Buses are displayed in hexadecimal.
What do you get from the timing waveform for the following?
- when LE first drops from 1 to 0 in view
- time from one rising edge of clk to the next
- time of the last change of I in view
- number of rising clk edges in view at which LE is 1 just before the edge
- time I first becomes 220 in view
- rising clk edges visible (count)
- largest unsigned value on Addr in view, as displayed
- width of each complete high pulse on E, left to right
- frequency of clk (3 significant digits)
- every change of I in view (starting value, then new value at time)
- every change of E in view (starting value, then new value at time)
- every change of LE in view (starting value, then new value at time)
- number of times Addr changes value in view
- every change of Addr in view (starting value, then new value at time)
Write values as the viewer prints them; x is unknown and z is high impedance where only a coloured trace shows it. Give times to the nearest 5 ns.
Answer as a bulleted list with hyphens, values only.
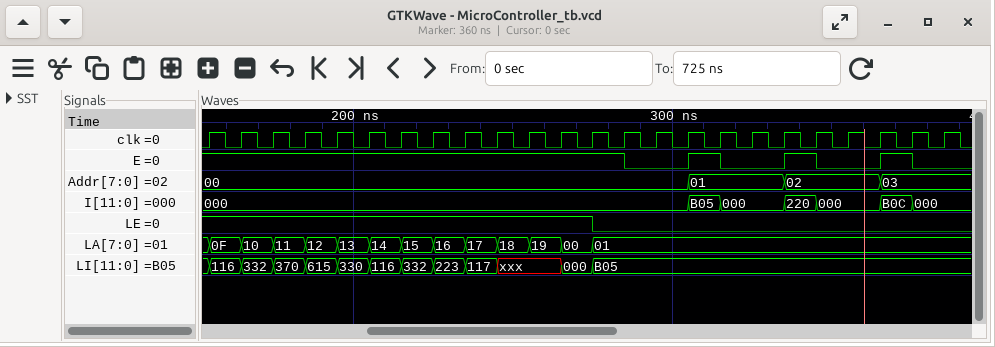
- 275 ns
- 10 ns
- 375 ns
- 13
- 335 ns
- 24
- 03
- 10 ns, 10 ns, 10 ns
- 100 MHz
- 000, B05 at 305 ns, 000 at 315 ns, 220 at 335 ns, 000 at 345 ns, B0C at 365 ns, 000 at 375 ns
- 1, 0 at 285 ns, 1 at 305 ns, 0 at 315 ns, 1 at 335 ns, 0 at 345 ns, 1 at 365 ns, 0 at 375 ns
- 1, 0 at 275 ns
- 3
- 00, 01 at 305 ns, 02 at 335 ns, 03 at 365 ns
